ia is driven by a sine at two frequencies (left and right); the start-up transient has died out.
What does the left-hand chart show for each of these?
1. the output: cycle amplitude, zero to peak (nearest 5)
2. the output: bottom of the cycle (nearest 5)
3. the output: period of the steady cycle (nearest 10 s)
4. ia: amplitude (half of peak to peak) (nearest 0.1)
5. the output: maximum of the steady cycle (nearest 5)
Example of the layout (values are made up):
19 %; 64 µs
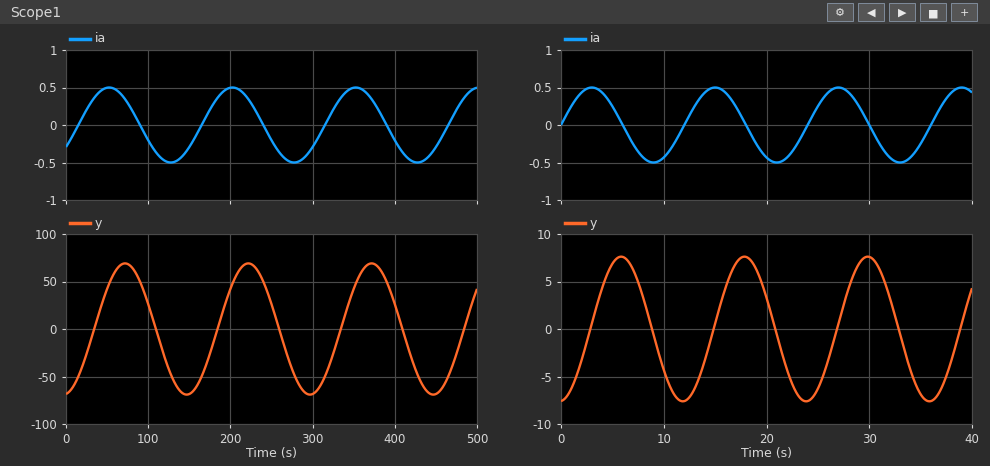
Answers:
70; -70; 150 s; 0.5; 70
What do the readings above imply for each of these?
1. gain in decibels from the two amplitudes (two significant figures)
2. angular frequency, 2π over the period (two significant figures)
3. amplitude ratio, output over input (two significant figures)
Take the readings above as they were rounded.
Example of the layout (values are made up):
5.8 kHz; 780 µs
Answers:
43 dB; 0.042 rad/s; 140
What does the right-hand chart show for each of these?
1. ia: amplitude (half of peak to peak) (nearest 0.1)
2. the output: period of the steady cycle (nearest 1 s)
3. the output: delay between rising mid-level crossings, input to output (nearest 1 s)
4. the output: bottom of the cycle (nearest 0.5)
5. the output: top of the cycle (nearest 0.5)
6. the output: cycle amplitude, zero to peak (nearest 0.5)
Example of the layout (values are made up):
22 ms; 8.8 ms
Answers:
0.5; 12 s; 3 s; -7.5; 7.5; 7.5
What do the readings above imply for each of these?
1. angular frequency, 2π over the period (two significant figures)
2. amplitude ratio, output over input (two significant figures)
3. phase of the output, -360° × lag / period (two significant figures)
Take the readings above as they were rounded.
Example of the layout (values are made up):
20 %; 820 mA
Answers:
0.52 rad/s; 15; -90°
